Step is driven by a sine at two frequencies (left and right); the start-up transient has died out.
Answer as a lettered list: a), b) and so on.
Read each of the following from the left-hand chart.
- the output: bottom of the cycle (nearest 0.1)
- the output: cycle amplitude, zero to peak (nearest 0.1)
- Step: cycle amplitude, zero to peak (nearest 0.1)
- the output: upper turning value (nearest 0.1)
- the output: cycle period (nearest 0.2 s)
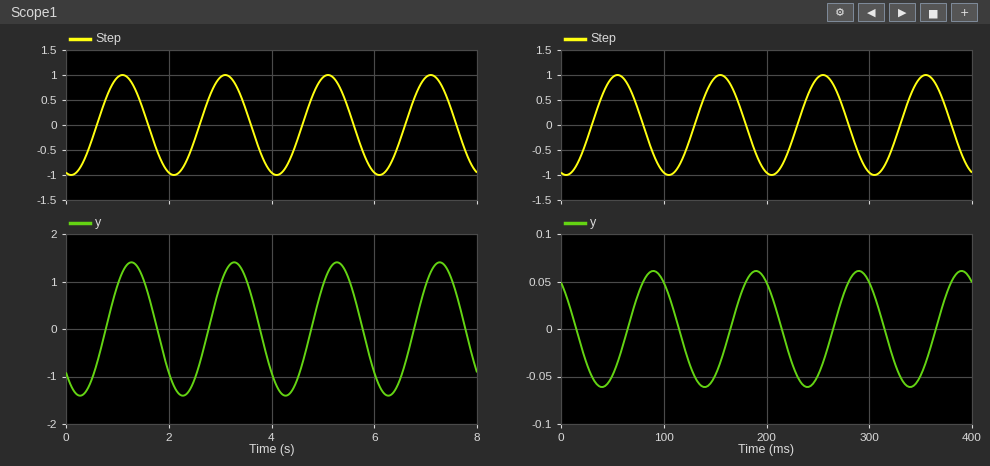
a) -1.4
b) 1.4
c) 1.0
d) 1.4
e) 2.0 s
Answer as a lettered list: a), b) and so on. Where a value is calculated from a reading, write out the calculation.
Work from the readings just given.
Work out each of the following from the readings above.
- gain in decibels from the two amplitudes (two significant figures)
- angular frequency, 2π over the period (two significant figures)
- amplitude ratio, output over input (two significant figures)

a) 20 log10(1.4 / 1) = 2.9 dB
b) 2π / 2 = 3.1 rad/s
c) 1.4 / 1 = 1.4
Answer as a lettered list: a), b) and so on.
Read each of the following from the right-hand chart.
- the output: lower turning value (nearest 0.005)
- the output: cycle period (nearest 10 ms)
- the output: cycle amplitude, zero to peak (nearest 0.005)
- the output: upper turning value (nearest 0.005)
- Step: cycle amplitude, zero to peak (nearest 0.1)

a) -0.060
b) 100 ms
c) 0.060
d) 0.060
e) 1.0
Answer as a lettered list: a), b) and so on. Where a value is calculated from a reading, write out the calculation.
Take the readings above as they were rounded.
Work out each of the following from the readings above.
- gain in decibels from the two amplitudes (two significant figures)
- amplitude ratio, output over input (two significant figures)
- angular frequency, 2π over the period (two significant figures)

a) 20 log10(0.06 / 1) = -24 dB
b) 0.06 / 1 = 0.060
c) 2π / 100 = 0.063 rad/ms
